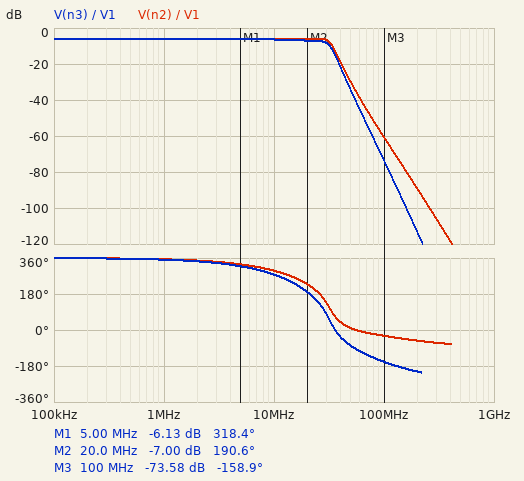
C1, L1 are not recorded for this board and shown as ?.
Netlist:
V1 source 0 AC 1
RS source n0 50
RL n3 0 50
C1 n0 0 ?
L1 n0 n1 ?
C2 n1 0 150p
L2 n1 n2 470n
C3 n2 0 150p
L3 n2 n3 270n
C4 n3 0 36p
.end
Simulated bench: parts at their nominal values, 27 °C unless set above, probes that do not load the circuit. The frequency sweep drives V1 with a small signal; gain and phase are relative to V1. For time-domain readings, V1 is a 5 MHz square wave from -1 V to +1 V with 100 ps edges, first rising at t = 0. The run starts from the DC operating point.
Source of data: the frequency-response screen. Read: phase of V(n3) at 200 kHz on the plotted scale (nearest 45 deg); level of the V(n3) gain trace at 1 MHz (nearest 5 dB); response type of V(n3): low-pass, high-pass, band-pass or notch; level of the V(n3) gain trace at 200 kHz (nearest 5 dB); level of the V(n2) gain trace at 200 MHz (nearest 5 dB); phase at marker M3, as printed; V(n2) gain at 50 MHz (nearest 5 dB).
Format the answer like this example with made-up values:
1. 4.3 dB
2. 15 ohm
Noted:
1. 360 deg
2. -5 dB
3. low-pass
4. -5 dB
5. -90 dB
6. -158.9 deg
7. -30 dB
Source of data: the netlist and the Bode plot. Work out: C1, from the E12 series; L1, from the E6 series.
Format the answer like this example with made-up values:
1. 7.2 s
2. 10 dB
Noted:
1. 22 pF
2. 680 nH
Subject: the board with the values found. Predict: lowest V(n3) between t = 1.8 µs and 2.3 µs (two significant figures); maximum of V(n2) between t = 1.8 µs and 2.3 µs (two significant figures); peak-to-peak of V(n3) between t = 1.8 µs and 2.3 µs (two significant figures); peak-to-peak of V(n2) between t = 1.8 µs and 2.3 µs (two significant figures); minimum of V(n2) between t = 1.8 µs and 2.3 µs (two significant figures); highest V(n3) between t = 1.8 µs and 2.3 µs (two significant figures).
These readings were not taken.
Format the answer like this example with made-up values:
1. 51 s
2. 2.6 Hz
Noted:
1. -600 mV
2. 630 mV
3. 1.2 V
4. 1.3 V
5. -630 mV
6. 600 mV
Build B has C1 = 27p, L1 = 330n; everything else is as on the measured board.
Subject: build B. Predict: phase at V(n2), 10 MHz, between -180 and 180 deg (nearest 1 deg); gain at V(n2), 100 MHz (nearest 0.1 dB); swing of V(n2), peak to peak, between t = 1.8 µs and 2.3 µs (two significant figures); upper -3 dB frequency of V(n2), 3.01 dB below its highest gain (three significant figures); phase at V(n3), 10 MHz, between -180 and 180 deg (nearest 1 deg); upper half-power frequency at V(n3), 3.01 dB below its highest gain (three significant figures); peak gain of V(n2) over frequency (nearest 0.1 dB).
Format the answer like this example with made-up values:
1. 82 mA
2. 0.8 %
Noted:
1. -52 deg
2. -54.2 dB
3. 1.4 V
4. 36.7 MHz
5. -72 deg
6. 35.7 MHz
7. -4.5 dB
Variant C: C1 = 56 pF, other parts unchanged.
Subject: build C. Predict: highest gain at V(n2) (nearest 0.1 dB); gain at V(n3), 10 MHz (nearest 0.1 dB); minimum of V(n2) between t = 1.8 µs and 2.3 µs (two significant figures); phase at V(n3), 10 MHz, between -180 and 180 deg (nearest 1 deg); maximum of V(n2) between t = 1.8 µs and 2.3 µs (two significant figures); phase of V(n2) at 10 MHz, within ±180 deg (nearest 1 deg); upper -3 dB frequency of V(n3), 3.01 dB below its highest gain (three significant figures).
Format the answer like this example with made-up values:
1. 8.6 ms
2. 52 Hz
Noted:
1. -5.9 dB
2. -6.3 dB
3. -650 mV
4. -87 deg
5. 650 mV
6. -67 deg
7. 31.6 MHz
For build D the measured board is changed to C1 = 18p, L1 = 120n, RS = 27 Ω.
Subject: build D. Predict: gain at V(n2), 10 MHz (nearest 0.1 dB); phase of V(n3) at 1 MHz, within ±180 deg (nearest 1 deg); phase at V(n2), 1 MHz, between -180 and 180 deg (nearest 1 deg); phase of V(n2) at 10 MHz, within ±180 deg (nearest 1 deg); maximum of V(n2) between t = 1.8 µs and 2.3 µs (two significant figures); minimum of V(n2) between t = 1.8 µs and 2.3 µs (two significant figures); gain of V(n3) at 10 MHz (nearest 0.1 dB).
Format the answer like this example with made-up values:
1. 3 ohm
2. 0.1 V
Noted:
1. -3.7 dB
2. -6 deg
3. -4 deg
4. -43 deg
5. 870 mV
6. -870 mV
7. -3.8 dB
